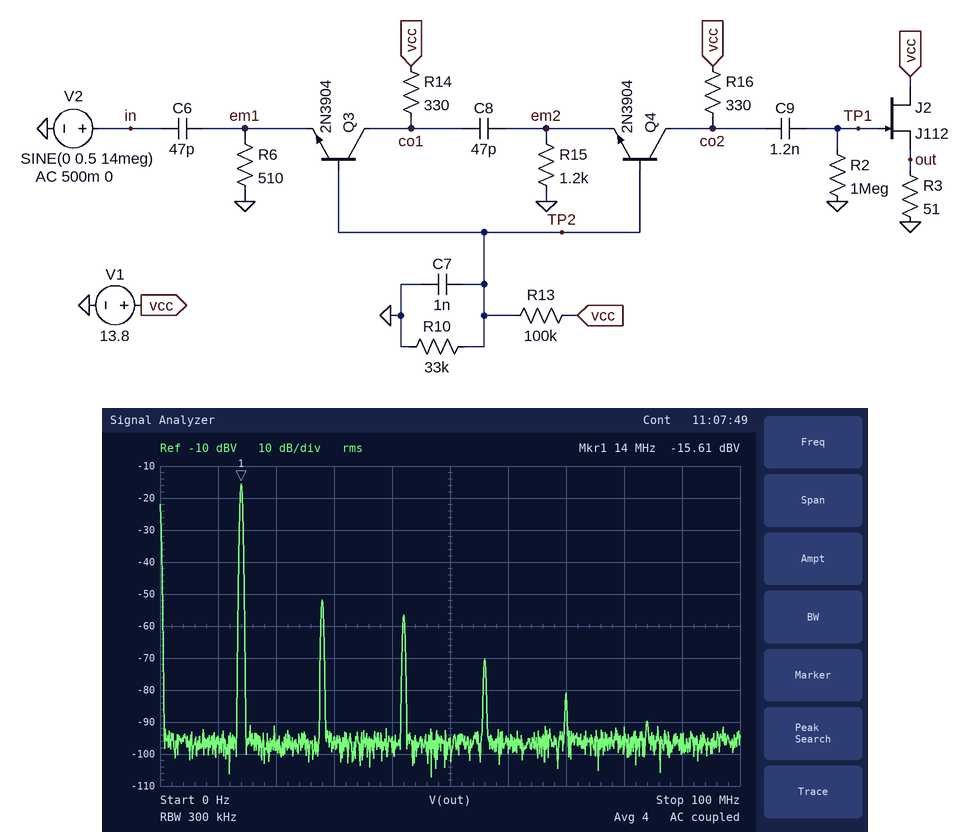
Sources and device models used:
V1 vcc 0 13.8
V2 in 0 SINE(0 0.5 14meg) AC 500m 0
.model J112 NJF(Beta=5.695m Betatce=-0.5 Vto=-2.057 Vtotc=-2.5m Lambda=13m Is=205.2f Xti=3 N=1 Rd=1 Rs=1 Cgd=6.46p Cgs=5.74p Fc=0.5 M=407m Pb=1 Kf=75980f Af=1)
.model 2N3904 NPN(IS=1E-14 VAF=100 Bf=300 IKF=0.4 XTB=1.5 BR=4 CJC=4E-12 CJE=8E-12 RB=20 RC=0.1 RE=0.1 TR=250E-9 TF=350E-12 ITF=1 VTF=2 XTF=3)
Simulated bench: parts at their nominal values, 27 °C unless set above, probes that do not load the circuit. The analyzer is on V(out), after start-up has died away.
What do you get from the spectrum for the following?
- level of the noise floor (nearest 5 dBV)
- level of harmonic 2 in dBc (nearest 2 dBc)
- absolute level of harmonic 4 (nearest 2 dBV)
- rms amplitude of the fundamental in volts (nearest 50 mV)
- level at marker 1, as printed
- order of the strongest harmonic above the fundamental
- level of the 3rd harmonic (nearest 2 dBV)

-95 dBV
-36 dBc
-70 dBV
150 mV
-15.61 dBV
2
-56 dBV
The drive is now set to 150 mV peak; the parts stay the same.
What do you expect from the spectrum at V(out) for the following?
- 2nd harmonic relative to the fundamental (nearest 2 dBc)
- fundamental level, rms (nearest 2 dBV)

-48 dBc
-26 dBV
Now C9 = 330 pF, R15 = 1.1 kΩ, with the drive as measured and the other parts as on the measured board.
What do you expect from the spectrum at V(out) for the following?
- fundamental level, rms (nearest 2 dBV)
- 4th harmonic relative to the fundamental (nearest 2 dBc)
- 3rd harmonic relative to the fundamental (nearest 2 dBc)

-16 dBV
-58 dBc
-42 dBc
